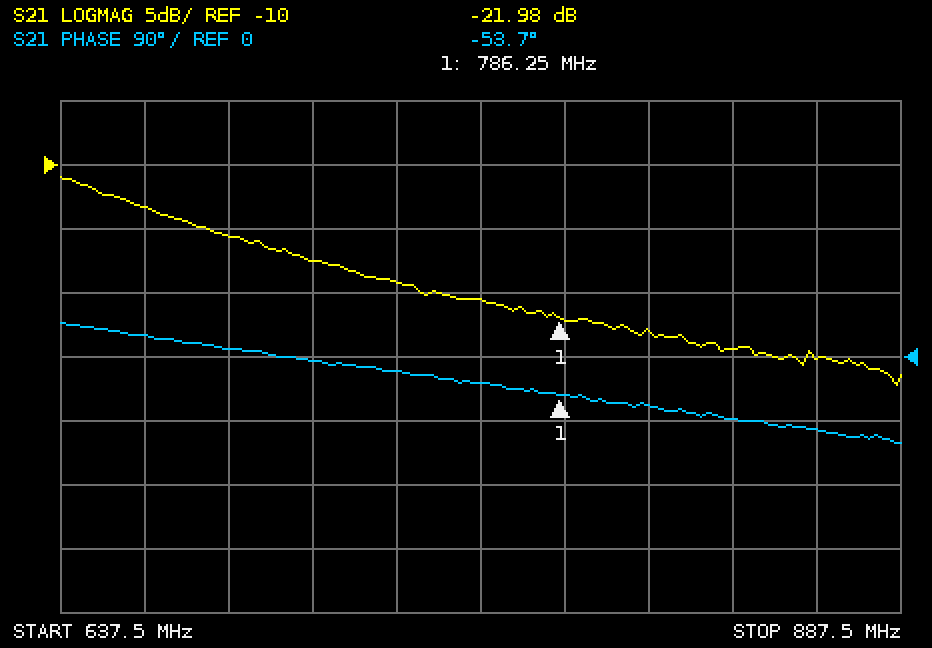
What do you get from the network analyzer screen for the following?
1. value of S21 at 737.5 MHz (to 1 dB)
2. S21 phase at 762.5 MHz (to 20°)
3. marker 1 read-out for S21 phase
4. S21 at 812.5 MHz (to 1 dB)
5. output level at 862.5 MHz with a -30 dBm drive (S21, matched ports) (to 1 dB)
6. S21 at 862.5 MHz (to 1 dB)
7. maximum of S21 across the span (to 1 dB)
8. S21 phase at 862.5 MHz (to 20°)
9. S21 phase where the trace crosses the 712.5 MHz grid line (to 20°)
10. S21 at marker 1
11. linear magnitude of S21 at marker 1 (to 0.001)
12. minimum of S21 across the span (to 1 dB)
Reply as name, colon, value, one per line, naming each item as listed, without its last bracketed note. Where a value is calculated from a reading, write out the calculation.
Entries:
value of S21 at 737.5 MHz: -19 dB
S21 phase at 762.5 MHz: -40°
marker 1 read-out for S21 phase: -53.7°
S21 at 812.5 MHz: -23 dB
output level at 862.5 MHz with a -30 dBm drive (S21, matched ports): -30 dBm + (-25 dB) = -55 dBm
S21 at 862.5 MHz: -25 dB
maximum of S21 across the span: -11 dB
S21 phase at 862.5 MHz: -100°
S21 phase where the trace crosses the 712.5 MHz grid line: 0°
S21 at marker 1: -21.98 dB
linear magnitude of S21 at marker 1: 10^(-21.98/20) ≈ 0.080
minimum of S21 across the span: -27 dB
